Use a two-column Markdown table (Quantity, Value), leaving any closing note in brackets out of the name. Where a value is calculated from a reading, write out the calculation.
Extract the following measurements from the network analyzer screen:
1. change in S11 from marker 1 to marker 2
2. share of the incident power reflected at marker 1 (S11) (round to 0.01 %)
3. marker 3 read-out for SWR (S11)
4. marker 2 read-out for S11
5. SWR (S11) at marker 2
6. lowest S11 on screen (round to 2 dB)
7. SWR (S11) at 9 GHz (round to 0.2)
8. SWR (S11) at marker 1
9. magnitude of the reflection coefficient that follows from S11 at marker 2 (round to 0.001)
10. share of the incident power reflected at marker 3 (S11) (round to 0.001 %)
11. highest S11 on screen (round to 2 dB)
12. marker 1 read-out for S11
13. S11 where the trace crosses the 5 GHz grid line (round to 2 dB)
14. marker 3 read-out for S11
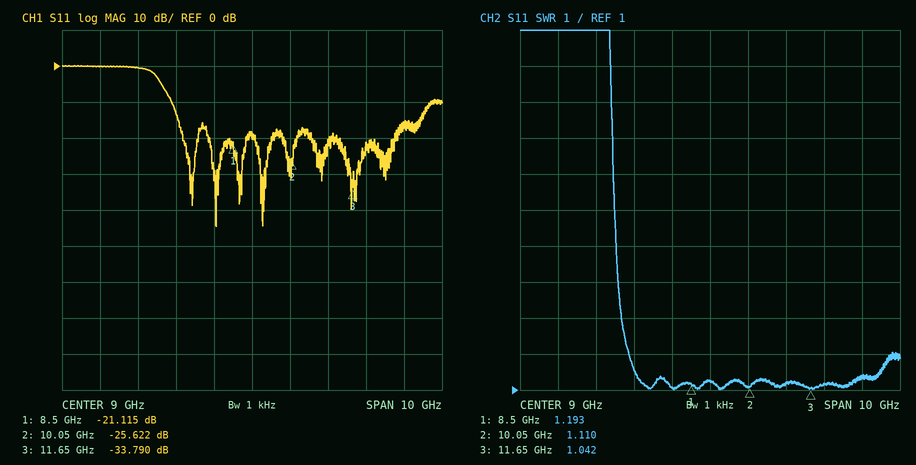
| Quantity | Value |
|---|---|
| change in S11 from marker 1 to marker 2 | -25.622 − (-21.115) = -4.507 dB |
| share of the incident power reflected at marker 1 (S11) | 10^(-21.115/10) ≈ 0.77 % |
| marker 3 read-out for SWR | 1.042 |
| marker 2 read-out for S11 | -25.622 dB |
| SWR (S11) at marker 2 | 1.110 |
| lowest S11 on screen | -44 dB |
| SWR (S11) at 9 GHz | 1.2 |
| SWR (S11) at marker 1 | 1.193 |
| magnitude of the reflection coefficient that follows from S11 at marker 2 | 10^(-25.622/20) ≈ 0.052 |
| share of the incident power reflected at marker 3 (S11) | 10^(-33.79/10) ≈ 0.042 % |
| highest S11 on screen | 0 dB |
| marker 1 read-out for S11 | -21.115 dB |
| S11 where the trace crosses the 5 GHz grid line | 0 dB |
| marker 3 read-out for S11 | -33.790 dB |
